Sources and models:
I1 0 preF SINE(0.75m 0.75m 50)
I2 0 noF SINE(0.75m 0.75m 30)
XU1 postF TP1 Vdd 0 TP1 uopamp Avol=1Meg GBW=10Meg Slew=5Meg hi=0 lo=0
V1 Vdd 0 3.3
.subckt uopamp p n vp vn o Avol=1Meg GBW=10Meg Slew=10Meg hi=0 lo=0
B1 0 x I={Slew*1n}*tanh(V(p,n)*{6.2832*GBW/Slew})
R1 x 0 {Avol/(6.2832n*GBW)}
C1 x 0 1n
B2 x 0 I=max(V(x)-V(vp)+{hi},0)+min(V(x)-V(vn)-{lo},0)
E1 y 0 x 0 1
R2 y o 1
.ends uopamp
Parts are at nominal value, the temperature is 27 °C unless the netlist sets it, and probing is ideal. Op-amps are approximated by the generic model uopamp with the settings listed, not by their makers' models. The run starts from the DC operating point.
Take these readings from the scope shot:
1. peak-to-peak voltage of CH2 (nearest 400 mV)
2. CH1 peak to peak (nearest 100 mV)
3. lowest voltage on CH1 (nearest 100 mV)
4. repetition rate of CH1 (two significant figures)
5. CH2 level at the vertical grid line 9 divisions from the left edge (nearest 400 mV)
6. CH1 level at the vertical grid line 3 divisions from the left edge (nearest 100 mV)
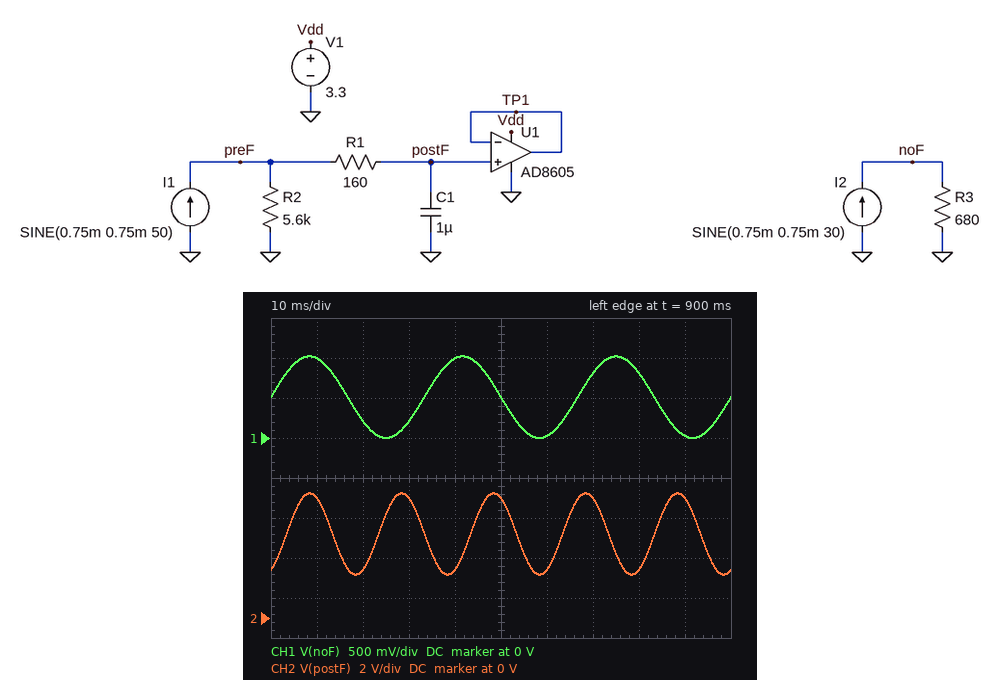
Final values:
4.0 V
1.0 V
0 V
30 Hz
6.0 V
200 mV
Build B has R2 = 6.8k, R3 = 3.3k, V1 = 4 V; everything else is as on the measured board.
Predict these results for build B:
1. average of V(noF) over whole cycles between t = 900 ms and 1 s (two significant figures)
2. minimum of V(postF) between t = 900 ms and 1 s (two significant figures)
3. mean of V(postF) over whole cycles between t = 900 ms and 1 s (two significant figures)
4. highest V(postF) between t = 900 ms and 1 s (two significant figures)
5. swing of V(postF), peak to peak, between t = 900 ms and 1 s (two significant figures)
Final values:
2.5 V
3.0 V
5.1 V
7.2 V
4.2 V
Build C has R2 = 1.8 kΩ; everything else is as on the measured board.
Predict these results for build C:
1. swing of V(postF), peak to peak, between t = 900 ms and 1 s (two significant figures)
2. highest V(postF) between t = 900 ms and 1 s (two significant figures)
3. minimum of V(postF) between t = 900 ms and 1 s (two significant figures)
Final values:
2.3 V
2.5 V
200 mV
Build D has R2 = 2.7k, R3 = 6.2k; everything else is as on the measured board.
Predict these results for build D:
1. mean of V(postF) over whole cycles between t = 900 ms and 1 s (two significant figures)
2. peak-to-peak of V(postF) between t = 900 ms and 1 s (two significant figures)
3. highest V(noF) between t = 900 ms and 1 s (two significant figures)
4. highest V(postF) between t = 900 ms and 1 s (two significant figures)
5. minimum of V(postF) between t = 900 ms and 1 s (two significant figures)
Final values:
2.0 V
3.0 V
9.3 V
3.5 V
520 mV
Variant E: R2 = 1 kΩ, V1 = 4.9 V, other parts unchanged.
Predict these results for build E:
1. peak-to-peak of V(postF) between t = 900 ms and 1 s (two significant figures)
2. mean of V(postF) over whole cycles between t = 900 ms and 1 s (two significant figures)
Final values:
1.4 V
750 mV
